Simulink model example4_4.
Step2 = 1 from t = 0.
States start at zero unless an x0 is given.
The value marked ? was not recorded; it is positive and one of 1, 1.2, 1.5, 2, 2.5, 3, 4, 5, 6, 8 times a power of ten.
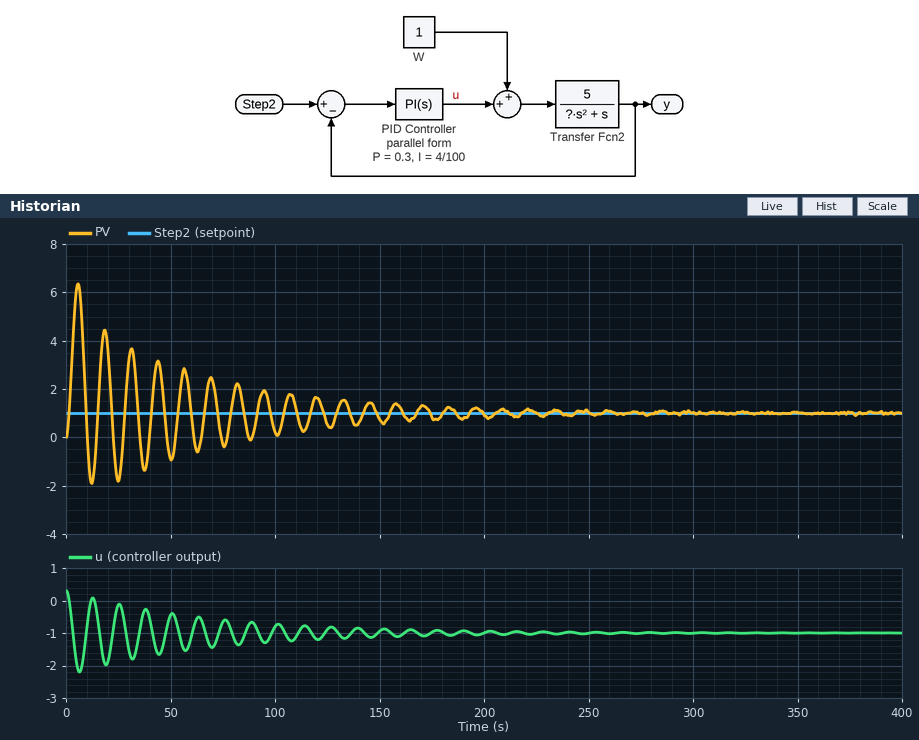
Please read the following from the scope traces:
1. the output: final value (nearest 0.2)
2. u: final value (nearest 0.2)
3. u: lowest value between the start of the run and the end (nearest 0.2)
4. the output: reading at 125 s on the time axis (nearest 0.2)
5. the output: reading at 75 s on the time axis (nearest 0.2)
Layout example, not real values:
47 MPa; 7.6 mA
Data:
1.0; -1.0; -2.2; 0.6; -0.2
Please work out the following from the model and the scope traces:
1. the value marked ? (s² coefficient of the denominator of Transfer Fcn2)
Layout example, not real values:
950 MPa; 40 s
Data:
6
